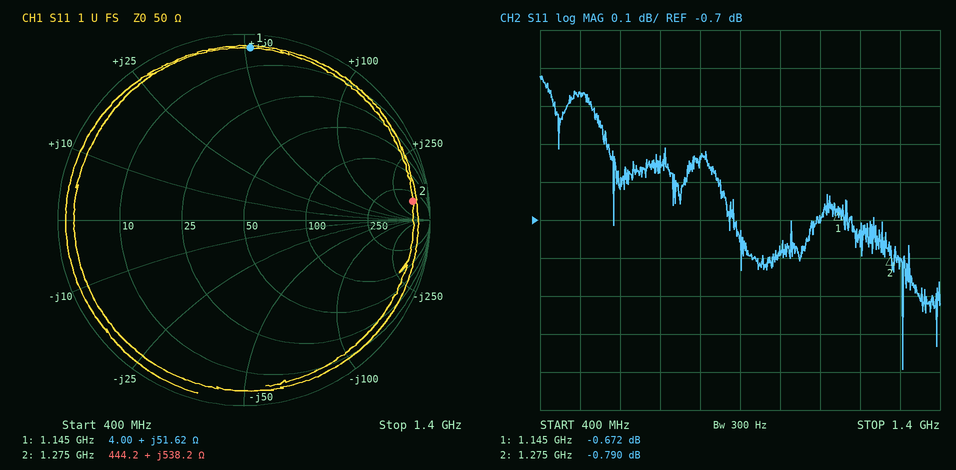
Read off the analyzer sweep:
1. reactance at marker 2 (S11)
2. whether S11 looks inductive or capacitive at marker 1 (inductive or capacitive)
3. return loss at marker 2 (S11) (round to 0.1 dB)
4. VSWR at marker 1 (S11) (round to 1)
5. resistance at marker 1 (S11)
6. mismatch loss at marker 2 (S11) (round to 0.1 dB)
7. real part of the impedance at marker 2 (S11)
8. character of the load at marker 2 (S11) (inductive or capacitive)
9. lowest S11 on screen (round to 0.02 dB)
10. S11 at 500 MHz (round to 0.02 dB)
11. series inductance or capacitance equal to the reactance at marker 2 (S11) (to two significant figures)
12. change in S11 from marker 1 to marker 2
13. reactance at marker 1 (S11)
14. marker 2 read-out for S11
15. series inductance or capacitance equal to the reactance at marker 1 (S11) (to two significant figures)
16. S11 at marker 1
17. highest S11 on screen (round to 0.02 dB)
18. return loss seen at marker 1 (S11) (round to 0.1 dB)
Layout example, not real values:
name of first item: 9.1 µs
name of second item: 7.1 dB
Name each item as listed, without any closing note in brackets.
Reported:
reactance at marker 2: +538.2 Ω
whether S11 looks inductive or capacitive at marker 1: inductive
return loss at marker 2 (S11): 0.8 dB
VSWR at marker 1 (S11): 26
resistance at marker 1: 4.00 Ω
mismatch loss at marker 2 (S11): 7.8 dB
real part of the impedance at marker 2: 444.2 Ω
character of the load at marker 2 (S11): inductive
lowest S11 on screen: -1.10 dB
S11 at 500 MHz: -0.36 dB
series inductance or capacitance equal to the reactance at marker 2 (S11): 67 nH
change in S11 from marker 1 to marker 2: -0.118 dB
reactance at marker 1: +51.62 Ω
marker 2 read-out for S11: -0.790 dB
series inductance or capacitance equal to the reactance at marker 1 (S11): 7.2 nH
S11 at marker 1: -0.672 dB
highest S11 on screen: -0.32 dB
return loss seen at marker 1 (S11): 0.7 dB
